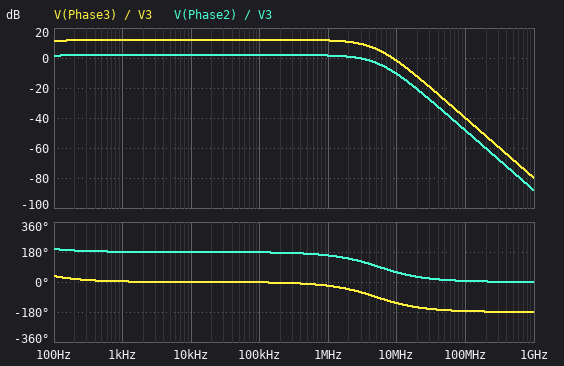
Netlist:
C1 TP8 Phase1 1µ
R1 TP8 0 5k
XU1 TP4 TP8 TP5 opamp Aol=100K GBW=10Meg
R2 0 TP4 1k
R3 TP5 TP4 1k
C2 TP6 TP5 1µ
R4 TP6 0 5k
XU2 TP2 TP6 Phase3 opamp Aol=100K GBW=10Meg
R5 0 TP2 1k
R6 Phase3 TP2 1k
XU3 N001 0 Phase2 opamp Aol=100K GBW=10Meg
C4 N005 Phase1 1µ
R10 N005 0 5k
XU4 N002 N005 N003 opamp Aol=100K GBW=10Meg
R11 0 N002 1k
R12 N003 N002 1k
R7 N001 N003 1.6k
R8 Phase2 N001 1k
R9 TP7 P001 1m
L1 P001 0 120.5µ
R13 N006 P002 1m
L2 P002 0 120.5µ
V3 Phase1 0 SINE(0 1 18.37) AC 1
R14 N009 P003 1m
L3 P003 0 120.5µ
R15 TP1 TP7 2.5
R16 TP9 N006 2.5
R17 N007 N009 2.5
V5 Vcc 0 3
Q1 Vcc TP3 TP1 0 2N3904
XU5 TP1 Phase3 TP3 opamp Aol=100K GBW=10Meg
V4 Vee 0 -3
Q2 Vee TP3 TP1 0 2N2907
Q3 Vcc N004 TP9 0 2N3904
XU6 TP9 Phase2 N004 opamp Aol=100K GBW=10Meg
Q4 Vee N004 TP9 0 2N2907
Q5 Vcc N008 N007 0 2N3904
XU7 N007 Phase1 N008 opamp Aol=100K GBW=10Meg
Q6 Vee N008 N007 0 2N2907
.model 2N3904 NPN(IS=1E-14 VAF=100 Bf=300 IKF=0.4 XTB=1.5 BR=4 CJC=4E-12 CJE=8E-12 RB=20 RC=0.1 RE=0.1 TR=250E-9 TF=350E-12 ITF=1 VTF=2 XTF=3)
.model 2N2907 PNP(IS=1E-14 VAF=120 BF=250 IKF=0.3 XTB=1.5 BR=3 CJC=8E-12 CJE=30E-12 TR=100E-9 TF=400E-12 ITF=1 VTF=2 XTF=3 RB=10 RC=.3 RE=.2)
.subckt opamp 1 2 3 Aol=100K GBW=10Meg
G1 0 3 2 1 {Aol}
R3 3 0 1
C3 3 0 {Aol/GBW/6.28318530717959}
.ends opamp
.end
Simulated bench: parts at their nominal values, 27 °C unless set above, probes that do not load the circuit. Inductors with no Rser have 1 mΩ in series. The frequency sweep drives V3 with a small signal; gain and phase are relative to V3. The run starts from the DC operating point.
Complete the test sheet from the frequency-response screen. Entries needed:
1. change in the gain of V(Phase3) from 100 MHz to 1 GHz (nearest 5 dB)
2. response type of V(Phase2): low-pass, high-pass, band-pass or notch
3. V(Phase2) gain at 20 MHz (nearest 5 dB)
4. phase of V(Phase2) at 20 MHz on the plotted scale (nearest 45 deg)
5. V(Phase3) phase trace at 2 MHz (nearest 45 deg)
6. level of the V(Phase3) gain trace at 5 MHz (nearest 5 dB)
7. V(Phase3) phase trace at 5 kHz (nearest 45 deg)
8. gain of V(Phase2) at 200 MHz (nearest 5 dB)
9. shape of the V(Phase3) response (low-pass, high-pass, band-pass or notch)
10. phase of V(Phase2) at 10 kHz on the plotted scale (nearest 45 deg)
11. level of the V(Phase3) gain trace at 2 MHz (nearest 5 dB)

-40 dB
low-pass
-20 dB
45 deg
-45 deg
5 dB
0 deg
-60 dB
low-pass
180 deg
10 dB
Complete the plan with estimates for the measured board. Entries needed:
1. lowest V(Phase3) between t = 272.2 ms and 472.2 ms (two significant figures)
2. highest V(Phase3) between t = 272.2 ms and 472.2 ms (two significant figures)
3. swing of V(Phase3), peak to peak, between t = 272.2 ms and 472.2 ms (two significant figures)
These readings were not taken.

-1.0 V
1.0 V
2.0 V
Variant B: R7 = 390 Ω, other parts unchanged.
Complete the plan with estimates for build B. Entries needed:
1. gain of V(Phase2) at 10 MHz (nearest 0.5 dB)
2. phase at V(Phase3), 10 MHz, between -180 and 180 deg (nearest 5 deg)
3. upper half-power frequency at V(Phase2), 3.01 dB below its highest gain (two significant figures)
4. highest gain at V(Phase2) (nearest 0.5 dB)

-4.0 dB
-125 deg
2.3 MHz
14.0 dB
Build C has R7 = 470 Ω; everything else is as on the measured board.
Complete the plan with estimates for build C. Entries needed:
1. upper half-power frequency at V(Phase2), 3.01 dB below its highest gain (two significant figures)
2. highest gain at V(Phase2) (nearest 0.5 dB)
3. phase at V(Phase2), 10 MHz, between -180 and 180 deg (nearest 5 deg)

2.5 MHz
12.5 dB
45 deg
